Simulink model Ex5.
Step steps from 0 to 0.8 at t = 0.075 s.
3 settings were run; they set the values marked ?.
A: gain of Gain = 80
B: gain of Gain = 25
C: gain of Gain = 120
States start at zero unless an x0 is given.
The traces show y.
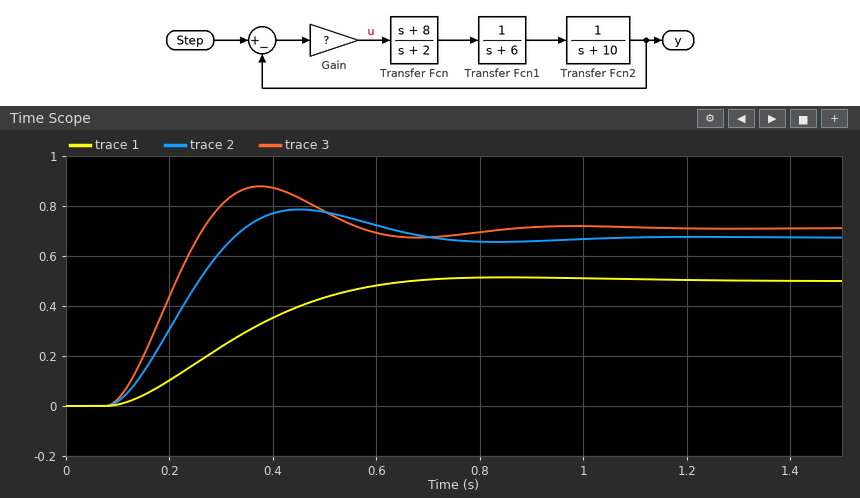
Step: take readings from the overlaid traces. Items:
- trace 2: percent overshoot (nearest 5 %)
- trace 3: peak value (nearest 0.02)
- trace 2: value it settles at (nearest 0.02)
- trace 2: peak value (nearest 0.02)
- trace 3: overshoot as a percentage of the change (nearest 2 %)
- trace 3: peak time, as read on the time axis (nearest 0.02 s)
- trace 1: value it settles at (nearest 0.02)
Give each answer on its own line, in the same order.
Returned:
15 %
0.88
0.68
0.78
24 %
0.38 s
0.50
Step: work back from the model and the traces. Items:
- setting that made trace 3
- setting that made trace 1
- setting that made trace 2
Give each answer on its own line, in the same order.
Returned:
C
B
A
